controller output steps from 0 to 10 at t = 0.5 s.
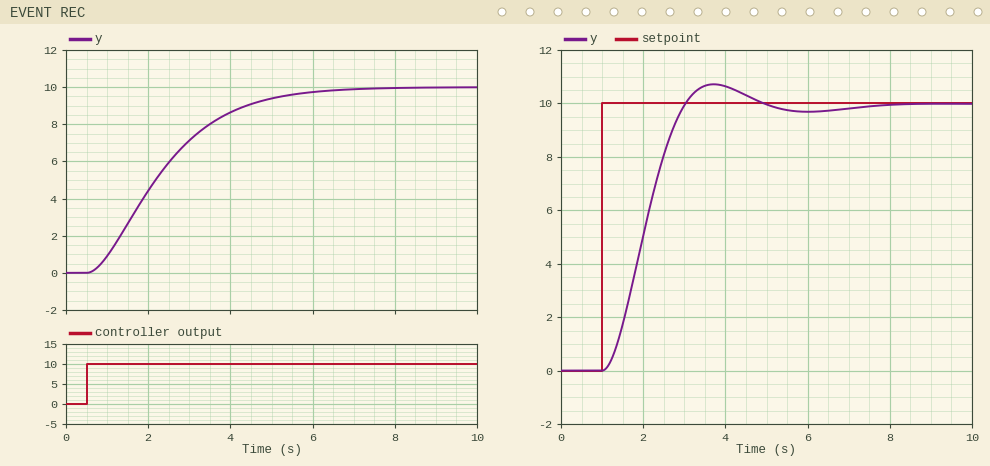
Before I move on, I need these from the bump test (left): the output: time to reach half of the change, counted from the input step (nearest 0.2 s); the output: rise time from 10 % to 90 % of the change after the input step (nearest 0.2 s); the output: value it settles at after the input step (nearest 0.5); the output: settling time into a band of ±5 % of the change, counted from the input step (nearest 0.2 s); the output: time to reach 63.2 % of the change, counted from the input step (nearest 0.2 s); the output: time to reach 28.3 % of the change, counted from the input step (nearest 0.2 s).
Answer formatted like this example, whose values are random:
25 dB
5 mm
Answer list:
1.6 s
3.4 s
10.0
4.8 s
2.2 s
1.0 s
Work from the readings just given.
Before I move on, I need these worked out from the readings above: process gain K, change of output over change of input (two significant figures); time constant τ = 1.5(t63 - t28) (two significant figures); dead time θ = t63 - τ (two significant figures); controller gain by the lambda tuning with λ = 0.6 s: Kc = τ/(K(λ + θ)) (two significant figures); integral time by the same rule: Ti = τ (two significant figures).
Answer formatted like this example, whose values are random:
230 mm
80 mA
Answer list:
1.0
1.8 s
0.40 s
1.8
1.8 s
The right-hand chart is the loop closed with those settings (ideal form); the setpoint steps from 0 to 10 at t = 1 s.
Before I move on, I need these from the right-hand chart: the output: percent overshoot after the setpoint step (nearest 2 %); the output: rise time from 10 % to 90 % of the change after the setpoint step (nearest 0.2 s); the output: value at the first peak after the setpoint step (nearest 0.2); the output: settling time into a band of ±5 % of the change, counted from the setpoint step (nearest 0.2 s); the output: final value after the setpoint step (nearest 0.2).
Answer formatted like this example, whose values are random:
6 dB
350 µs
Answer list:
8 %
1.4 s
10.8
3.2 s
10.0
